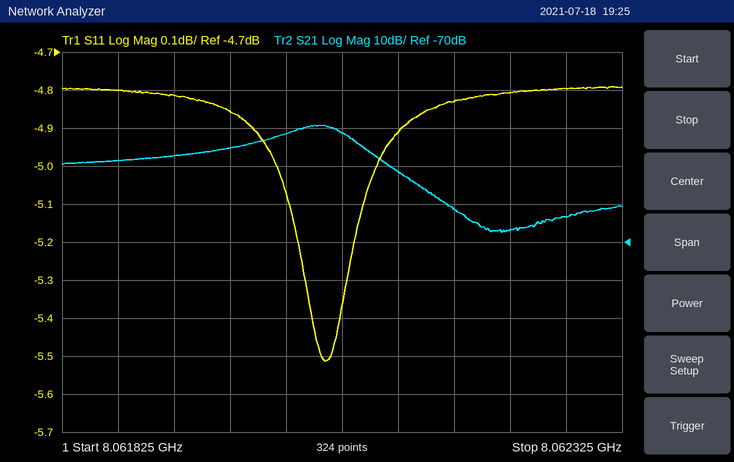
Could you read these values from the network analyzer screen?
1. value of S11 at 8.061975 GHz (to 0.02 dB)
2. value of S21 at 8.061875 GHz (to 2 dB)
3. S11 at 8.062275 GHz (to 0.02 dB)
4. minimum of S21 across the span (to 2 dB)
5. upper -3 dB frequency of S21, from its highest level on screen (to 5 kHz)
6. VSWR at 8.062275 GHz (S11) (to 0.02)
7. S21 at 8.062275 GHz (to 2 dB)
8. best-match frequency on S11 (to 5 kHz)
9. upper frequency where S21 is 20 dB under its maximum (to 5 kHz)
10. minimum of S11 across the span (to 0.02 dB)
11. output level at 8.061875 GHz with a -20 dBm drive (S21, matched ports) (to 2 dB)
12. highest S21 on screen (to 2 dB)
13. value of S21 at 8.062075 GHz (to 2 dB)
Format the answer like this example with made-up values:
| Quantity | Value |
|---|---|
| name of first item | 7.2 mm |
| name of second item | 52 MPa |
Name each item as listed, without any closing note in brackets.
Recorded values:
| Quantity | Value |
|---|---|
| value of S11 at 8.061975 GHz | -4.86 dB |
| value of S21 at 8.061875 GHz | -48 dB |
| S11 at 8.062275 GHz | -4.80 dB |
| minimum of S21 across the span | -68 dB |
| upper -3 dB frequency of S21, from its highest level on screen | 8.062080 GHz |
| VSWR at 8.062275 GHz (S11) | 3.72 |
| S21 at 8.062275 GHz | -64 dB |
| best-match frequency on S11 | 8.062060 GHz |
| upper frequency where S21 is 20 dB under its maximum | 8.062165 GHz |
| minimum of S11 across the span | -5.52 dB |
| output level at 8.061875 GHz with a -20 dBm drive (S21, matched ports) | -68 dBm |
| highest S21 on screen | -40 dB |
| value of S21 at 8.062075 GHz | -42 dB |
